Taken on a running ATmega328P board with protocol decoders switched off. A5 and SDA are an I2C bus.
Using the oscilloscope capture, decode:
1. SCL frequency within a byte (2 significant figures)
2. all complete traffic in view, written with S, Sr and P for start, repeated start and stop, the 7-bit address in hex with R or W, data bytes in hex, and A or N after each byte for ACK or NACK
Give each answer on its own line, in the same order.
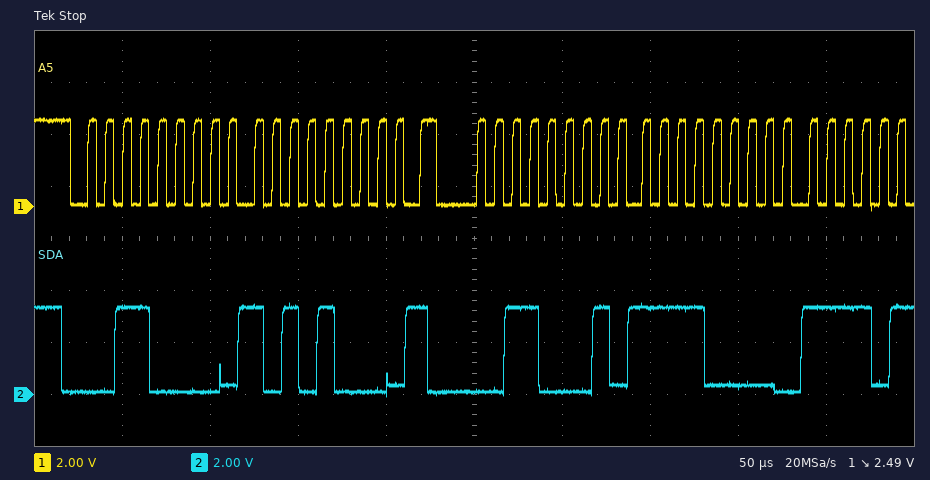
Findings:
100 kHz
S 18W A A8 A Sr 18R A F0 A
